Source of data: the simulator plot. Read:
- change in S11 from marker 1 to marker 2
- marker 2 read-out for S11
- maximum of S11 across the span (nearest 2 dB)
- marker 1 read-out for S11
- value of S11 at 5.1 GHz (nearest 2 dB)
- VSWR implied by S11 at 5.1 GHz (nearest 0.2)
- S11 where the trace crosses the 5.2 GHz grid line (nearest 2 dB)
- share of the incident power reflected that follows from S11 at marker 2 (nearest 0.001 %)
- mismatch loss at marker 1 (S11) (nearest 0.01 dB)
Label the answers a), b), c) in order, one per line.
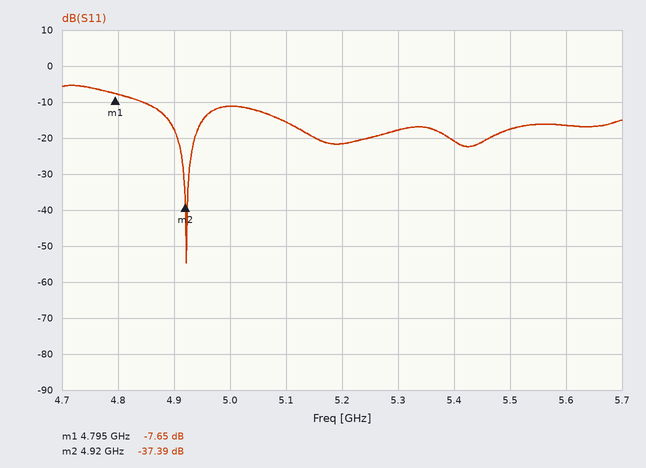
a) -29.74 dB
b) -37.39 dB
c) -6 dB
d) -7.65 dB
e) -16 dB
f) 1.4
g) -22 dB
h) 0.018 %
i) 0.82 dB
